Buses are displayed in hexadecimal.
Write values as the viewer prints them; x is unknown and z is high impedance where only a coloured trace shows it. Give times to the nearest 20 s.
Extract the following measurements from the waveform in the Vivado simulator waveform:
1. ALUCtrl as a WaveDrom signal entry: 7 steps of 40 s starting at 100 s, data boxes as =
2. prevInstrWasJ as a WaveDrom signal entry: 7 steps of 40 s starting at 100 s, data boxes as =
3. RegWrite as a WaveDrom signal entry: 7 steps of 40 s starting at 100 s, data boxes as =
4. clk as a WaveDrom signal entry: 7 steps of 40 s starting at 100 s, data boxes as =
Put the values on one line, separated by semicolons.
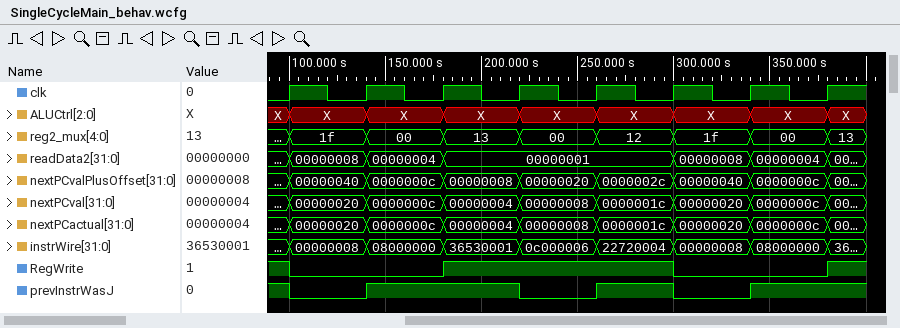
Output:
{name: 'ALUCtrl', wave: '==x====', data: 'X X X X X X'}; {name: 'prevInstrWasJ', wave: '01.0101'}; {name: 'RegWrite', wave: '0.1..0.'}; {name: 'clk', wave: 'p......'}
